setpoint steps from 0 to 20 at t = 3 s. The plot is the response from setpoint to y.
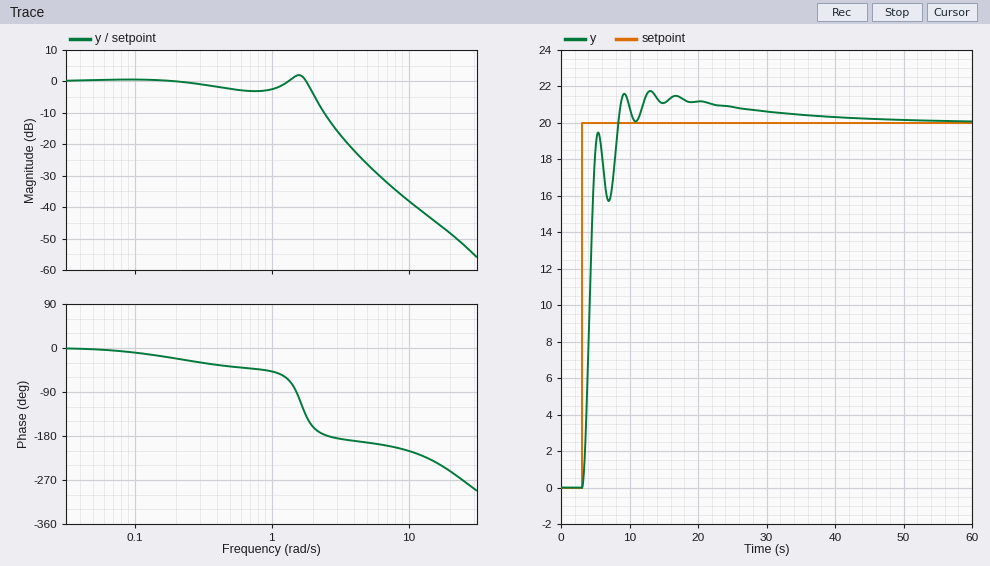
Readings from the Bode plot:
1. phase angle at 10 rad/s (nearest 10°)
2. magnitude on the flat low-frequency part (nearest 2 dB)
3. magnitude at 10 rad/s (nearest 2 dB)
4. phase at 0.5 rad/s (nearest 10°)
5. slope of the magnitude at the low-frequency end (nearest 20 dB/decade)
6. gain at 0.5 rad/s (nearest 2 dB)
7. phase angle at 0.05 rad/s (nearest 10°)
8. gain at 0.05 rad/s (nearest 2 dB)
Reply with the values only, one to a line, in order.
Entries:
-210°
0 dB
-38 dB
-40°
0 dB/decade
-2 dB
0°
0 dB
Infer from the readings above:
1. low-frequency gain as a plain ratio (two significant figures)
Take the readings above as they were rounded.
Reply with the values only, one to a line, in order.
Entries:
1.0
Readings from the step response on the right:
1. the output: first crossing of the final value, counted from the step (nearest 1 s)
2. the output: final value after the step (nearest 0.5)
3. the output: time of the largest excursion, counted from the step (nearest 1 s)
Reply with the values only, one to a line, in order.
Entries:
5 s
20.0
10 s
